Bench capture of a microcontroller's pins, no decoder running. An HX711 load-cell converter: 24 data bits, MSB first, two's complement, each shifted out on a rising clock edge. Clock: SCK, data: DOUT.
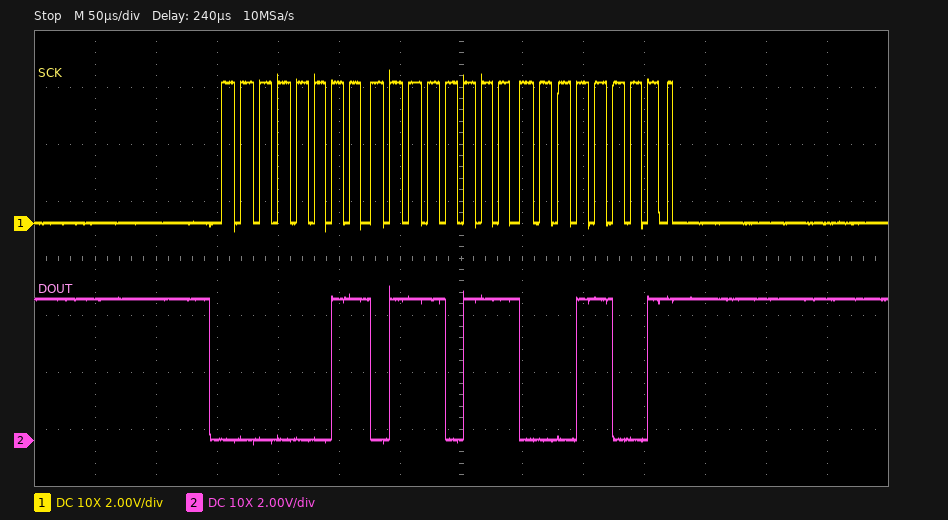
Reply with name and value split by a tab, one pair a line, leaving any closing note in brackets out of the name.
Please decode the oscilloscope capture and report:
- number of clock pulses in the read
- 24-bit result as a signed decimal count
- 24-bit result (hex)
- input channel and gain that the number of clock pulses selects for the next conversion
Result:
number of clock pulses in the read	25
24-bit result as a signed decimal count	227097
24-bit result	0x037719
input channel and gain that the number of clock pulses selects for the next conversion	channel A, gain 128
